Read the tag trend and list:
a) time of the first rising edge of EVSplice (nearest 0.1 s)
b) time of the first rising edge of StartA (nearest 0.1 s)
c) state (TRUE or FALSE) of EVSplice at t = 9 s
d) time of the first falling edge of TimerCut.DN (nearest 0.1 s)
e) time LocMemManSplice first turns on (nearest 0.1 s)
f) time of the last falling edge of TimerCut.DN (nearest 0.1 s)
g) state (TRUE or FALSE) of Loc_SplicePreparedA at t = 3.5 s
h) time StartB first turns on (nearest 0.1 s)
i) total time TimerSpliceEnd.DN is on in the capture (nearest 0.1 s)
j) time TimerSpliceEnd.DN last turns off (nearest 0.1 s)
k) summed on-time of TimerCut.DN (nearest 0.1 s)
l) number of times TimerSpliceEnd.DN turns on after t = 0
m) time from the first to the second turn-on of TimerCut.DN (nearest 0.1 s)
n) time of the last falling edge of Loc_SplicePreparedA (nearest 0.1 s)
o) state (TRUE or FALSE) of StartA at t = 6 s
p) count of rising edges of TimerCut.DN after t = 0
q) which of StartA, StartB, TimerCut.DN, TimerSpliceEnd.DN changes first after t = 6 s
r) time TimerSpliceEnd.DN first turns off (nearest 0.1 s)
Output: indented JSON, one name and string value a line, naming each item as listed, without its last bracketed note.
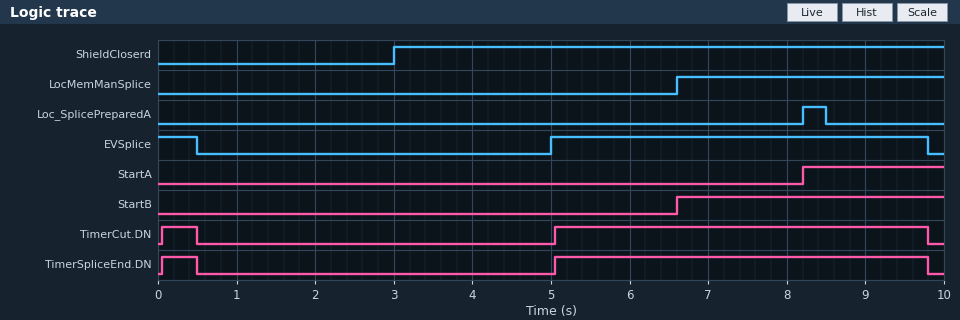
{
  "time of the first rising edge of EVSplice": "5.0 s",
  "time of the first rising edge of StartA": "8.2 s",
  "state (TRUE or FALSE) of EVSplice at t = 9 s": "TRUE",
  "time of the first falling edge of TimerCut.DN": "0.5 s",
  "time LocMemManSplice first turns on": "6.6 s",
  "time of the last falling edge of TimerCut.DN": "9.8 s",
  "state (TRUE or FALSE) of Loc_SplicePreparedA at t = 3.5 s": "FALSE",
  "time StartB first turns on": "6.6 s",
  "total time TimerSpliceEnd.DN is on in the capture": "5.2 s",
  "time TimerSpliceEnd.DN last turns off": "9.8 s",
  "summed on-time of TimerCut.DN": "5.2 s",
  "number of times TimerSpliceEnd.DN turns on after t = 0": "2",
  "time from the first to the second turn-on of TimerCut.DN": "5.0 s",
  "time of the last falling edge of Loc_SplicePreparedA": "8.5 s",
  "state (TRUE or FALSE) of StartA at t = 6 s": "FALSE",
  "count of rising edges of TimerCut.DN after t = 0": "2",
  "which of StartA, StartB, TimerCut.DN, TimerSpliceEnd.DN changes first after t = 6 s": "StartB",
  "time TimerSpliceEnd.DN first turns off": "0.5 s"
}
